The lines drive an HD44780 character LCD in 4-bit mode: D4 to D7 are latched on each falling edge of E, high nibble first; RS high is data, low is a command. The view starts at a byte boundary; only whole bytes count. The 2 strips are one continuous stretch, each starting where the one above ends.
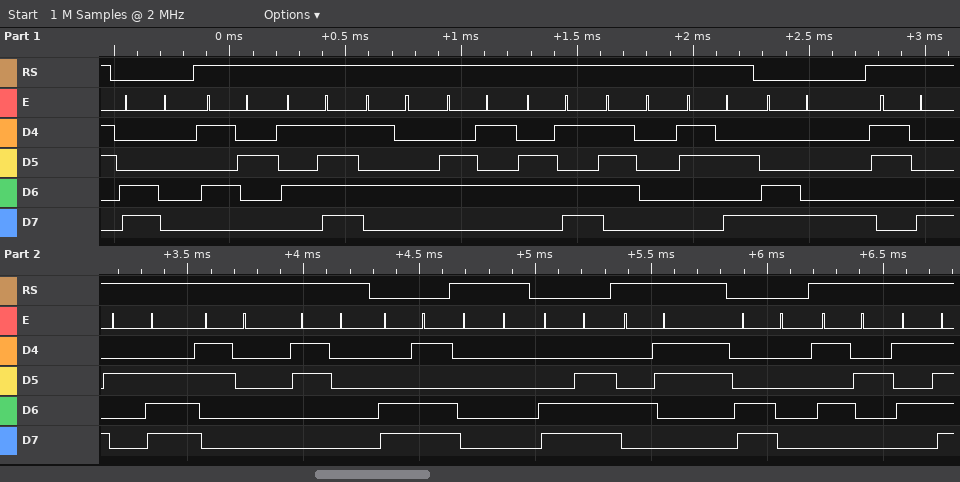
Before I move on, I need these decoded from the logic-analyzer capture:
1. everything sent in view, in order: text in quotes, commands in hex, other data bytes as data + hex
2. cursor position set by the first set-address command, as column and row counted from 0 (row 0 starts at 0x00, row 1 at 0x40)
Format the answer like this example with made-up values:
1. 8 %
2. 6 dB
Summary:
1. 0xC0 "R_Temp:" 0xC8 "8.00" 0xCD data 00 0xCE "C" 0xC0 "R_"
2. column 0, row 1
